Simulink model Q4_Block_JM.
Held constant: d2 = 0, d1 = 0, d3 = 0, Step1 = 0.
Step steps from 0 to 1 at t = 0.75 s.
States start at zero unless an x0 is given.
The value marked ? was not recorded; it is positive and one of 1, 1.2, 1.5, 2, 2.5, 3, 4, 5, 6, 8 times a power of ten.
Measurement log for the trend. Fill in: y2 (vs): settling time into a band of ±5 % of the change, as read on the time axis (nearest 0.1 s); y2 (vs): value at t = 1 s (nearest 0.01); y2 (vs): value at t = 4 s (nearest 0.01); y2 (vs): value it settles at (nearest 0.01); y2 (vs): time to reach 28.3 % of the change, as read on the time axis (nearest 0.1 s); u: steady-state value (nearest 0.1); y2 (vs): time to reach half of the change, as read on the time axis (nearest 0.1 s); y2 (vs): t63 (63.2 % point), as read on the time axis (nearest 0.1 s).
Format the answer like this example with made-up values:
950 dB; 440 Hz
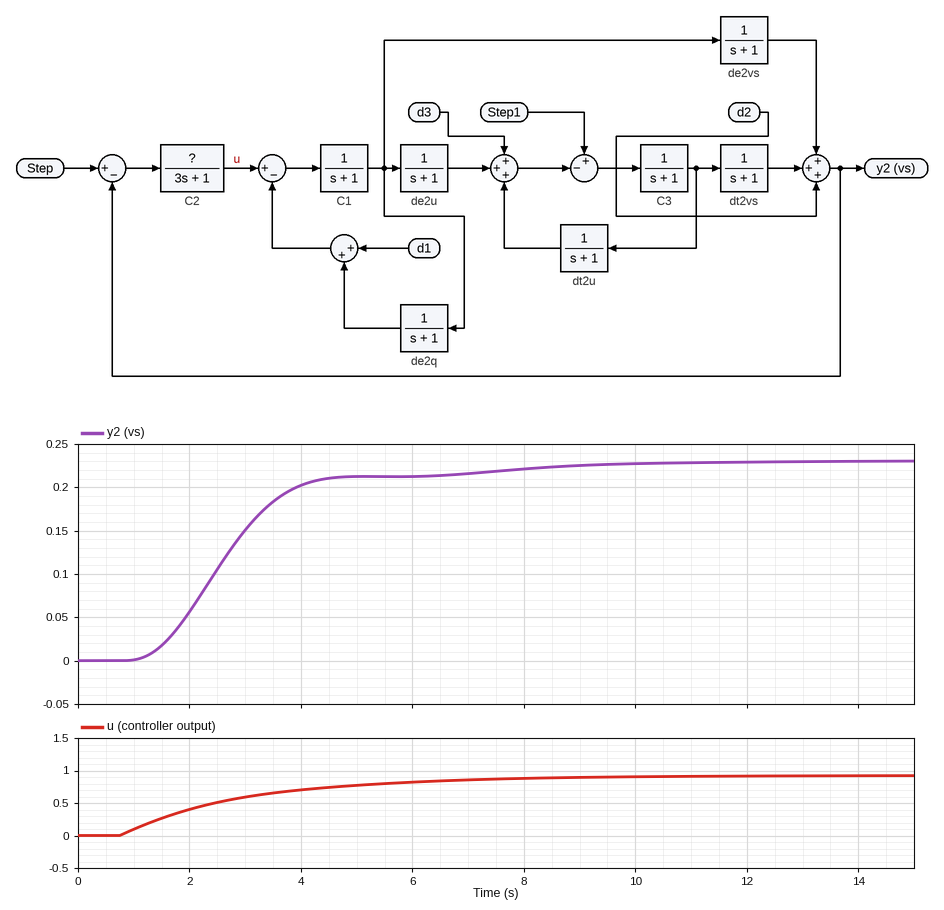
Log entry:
7.6 s; 0.00; 0.20; 0.23; 2.1 s; 0.9; 2.6 s; 2.9 s
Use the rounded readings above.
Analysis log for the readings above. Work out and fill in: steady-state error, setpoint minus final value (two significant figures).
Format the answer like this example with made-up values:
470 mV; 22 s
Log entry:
0.77
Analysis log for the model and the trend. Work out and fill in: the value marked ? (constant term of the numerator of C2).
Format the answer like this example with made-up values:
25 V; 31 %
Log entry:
1.2
